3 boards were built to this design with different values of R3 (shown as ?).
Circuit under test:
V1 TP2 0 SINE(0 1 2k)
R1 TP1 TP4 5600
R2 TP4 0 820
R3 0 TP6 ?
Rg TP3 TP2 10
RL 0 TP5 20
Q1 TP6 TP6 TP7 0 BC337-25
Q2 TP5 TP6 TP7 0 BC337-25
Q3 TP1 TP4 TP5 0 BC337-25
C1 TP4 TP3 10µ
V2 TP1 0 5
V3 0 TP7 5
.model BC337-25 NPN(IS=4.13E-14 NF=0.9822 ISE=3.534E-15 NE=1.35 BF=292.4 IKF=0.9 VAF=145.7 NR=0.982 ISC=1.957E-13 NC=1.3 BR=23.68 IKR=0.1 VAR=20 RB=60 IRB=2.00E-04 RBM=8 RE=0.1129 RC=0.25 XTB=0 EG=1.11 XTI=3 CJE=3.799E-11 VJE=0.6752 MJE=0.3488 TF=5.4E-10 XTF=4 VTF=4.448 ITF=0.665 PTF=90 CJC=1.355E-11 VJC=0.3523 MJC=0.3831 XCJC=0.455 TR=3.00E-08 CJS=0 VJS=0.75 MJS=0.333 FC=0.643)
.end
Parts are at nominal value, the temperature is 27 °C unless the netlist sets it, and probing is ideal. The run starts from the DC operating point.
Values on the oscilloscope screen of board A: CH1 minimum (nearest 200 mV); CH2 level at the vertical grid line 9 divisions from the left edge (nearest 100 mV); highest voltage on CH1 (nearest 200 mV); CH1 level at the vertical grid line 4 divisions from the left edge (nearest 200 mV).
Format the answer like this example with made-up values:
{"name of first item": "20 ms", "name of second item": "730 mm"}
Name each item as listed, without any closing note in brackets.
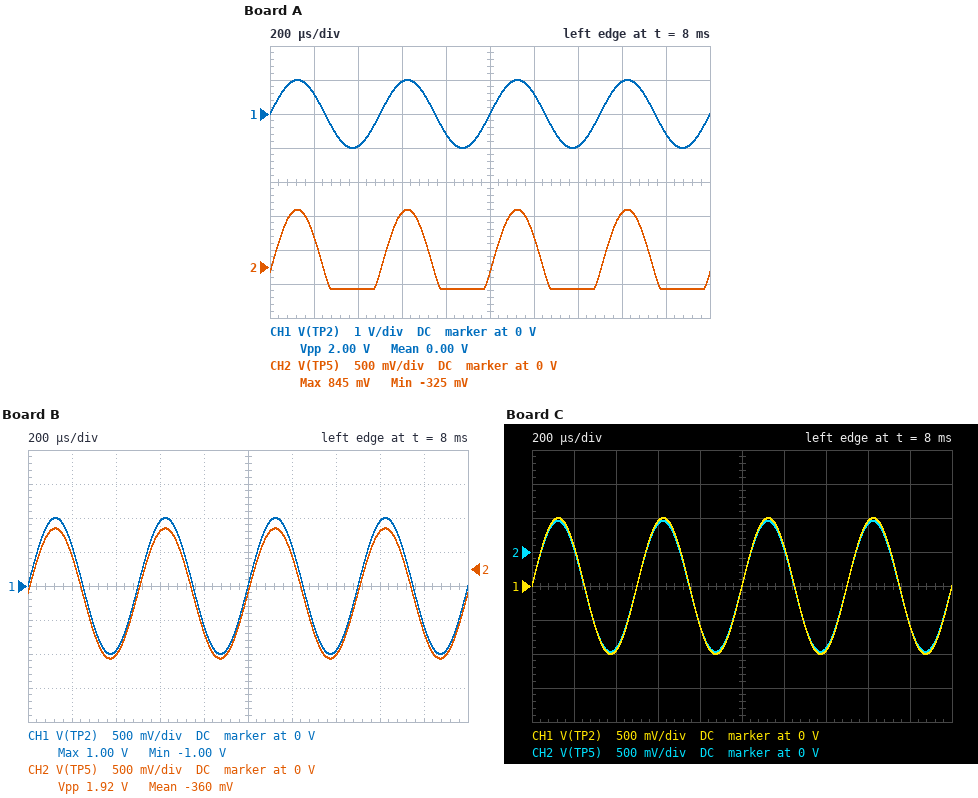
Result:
{"CH1 minimum": "-1.0 V", "CH2 level at the vertical grid line 9 divisions from the left edge": "-300 mV", "highest voltage on CH1": "1.0 V", "CH1 level at the vertical grid line 4 divisions from the left edge": "-600 mV"}
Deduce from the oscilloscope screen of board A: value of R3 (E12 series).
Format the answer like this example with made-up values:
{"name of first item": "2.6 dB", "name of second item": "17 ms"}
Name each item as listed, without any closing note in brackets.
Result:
{"value of R3": "270 Ω"}
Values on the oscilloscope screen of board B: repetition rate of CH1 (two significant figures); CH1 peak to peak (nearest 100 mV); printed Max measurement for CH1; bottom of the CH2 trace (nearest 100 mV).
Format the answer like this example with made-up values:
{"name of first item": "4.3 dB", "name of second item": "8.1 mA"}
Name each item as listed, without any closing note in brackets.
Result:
{"repetition rate of CH1": "2.0 kHz", "CH1 peak to peak": "2.0 V", "printed Max measurement for CH1": "1.00 V", "bottom of the CH2 trace": "-1.3 V"}
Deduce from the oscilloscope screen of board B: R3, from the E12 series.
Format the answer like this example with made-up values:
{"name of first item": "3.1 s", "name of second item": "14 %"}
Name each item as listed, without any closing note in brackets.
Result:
{"R3, from the E12 series": "39 Ω"}
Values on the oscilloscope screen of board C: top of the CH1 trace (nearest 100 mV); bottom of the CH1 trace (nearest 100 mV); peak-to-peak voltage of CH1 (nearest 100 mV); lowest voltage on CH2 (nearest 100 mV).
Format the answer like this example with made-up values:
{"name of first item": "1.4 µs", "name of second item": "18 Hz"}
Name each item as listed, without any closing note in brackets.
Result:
{"top of the CH1 trace": "1.0 V", "bottom of the CH1 trace": "-1.0 V", "peak-to-peak voltage of CH1": "2.0 V", "lowest voltage on CH2": "-1.5 V"}
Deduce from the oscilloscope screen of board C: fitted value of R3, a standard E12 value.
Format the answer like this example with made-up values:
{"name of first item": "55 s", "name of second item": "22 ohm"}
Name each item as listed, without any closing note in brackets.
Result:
{"fitted value of R3, a standard E12 value": "27 Ω"}
